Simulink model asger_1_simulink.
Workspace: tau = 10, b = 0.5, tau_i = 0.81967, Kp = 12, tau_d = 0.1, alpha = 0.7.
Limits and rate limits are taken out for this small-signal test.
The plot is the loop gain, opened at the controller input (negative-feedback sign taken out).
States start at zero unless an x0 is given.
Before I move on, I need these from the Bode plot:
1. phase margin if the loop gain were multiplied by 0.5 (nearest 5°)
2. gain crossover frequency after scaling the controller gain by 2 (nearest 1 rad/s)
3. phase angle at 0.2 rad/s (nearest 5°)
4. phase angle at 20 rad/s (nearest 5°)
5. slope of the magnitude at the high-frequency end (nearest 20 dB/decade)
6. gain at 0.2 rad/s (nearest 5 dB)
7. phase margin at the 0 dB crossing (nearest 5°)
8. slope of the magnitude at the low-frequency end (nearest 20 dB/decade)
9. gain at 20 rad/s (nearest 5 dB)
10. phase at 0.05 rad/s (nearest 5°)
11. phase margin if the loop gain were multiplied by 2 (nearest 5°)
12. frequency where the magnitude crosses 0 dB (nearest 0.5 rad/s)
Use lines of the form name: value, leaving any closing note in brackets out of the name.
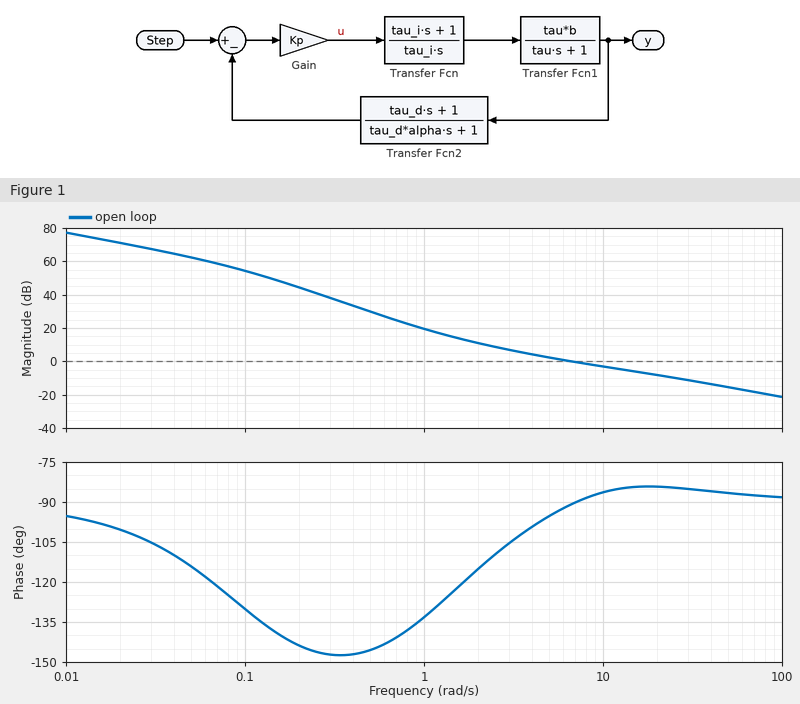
phase margin if the loop gain were multiplied by 0.5: 75°
gain crossover frequency after scaling the controller gain by 2: 15 rad/s
phase angle at 0.2 rad/s: -145°
phase angle at 20 rad/s: -85°
slope of the magnitude at the high-frequency end: -20 dB/decade
gain at 0.2 rad/s: 45 dB
phase margin at the 0 dB crossing: 90°
slope of the magnitude at the low-frequency end: -20 dB/decade
gain at 20 rad/s: -10 dB
phase at 0.05 rad/s: -115°
phase margin if the loop gain were multiplied by 2: 95°
frequency where the magnitude crosses 0 dB: 6.5 rad/s
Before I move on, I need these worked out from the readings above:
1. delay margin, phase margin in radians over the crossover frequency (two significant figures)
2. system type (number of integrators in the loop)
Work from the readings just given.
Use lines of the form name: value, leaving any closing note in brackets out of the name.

delay margin, phase margin in radians over the crossover frequency: 0.24 s
system type: 1
